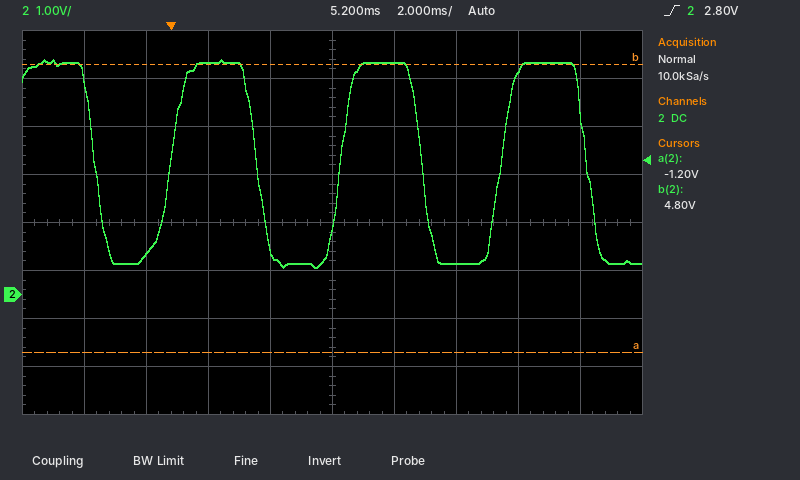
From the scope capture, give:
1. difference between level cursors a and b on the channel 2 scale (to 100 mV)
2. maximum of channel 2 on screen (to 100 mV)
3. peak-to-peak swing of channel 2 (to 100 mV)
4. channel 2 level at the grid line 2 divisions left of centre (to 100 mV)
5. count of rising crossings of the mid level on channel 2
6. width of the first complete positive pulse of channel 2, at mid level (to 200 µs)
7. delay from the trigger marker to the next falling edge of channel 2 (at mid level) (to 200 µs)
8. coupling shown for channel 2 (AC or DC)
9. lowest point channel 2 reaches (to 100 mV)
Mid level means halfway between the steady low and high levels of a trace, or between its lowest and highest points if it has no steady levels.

6.0 V
4.9 V
4.3 V
4.8 V
3
2.8 ms
2.8 ms
DC
600 mV
